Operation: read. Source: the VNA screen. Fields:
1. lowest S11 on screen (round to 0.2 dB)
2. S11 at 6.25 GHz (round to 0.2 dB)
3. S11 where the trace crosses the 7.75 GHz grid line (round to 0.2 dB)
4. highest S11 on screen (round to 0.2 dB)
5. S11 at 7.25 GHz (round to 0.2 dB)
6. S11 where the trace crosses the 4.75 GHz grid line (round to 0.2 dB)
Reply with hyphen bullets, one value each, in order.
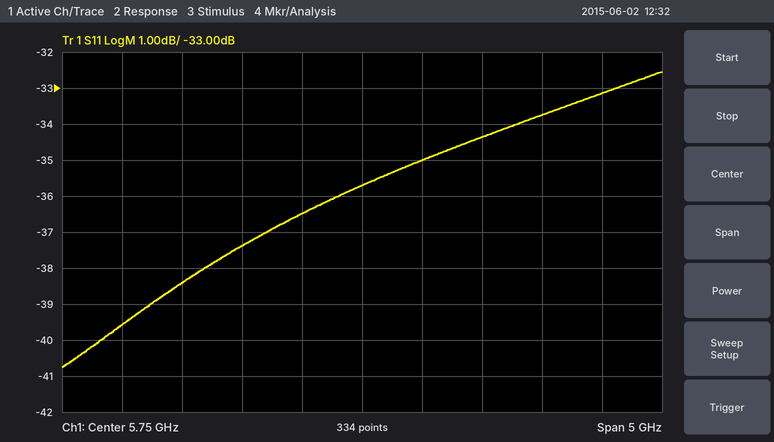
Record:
- -40.8 dB
- -35.0 dB
- -33.2 dB
- -32.6 dB
- -33.8 dB
- -37.4 dB
